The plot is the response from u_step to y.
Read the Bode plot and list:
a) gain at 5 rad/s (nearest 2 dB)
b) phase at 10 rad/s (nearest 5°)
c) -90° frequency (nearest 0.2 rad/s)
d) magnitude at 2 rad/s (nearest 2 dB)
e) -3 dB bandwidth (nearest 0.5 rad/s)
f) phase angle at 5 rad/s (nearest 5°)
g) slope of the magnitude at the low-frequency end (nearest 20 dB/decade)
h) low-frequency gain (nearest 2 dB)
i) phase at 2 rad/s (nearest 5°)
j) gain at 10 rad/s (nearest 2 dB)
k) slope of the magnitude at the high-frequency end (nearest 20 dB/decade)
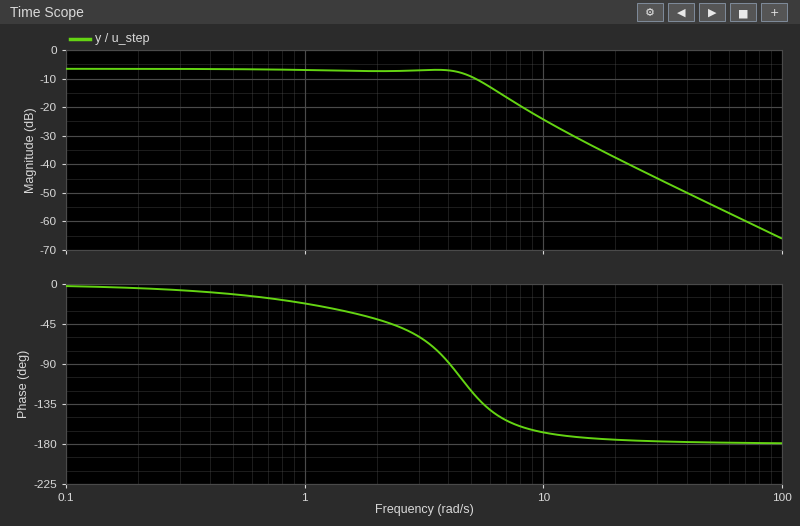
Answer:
-10 dB
-165°
4.0 rad/s
-8 dB
5.0 rad/s
-120°
0 dB/decade
-6 dB
-40°
-24 dB
-40 dB/decade
